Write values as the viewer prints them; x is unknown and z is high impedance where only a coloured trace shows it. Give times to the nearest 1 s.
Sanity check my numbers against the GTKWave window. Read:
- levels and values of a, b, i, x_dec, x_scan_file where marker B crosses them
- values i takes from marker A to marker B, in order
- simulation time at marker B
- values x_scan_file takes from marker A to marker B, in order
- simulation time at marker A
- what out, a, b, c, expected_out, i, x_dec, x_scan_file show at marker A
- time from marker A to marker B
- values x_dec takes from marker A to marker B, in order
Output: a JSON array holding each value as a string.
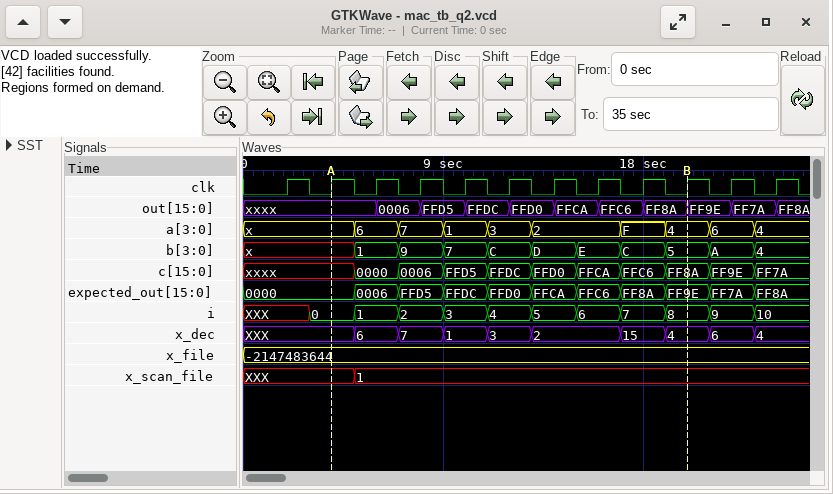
["a=4, b=5, i=8, x_dec=4, x_scan_file=1", "0, 1, 2, 3, 4, 5, 6, 7, 8", "20 s", "XXX, 1", "4 s", "out=xxxx, a=x, b=x, c=xxxx, expected_out=0000, i=0, x_dec=XXX, x_scan_file=XXX", "16 s", "XXX, 6, 7, 1, 3, 2, 15, 4"]
